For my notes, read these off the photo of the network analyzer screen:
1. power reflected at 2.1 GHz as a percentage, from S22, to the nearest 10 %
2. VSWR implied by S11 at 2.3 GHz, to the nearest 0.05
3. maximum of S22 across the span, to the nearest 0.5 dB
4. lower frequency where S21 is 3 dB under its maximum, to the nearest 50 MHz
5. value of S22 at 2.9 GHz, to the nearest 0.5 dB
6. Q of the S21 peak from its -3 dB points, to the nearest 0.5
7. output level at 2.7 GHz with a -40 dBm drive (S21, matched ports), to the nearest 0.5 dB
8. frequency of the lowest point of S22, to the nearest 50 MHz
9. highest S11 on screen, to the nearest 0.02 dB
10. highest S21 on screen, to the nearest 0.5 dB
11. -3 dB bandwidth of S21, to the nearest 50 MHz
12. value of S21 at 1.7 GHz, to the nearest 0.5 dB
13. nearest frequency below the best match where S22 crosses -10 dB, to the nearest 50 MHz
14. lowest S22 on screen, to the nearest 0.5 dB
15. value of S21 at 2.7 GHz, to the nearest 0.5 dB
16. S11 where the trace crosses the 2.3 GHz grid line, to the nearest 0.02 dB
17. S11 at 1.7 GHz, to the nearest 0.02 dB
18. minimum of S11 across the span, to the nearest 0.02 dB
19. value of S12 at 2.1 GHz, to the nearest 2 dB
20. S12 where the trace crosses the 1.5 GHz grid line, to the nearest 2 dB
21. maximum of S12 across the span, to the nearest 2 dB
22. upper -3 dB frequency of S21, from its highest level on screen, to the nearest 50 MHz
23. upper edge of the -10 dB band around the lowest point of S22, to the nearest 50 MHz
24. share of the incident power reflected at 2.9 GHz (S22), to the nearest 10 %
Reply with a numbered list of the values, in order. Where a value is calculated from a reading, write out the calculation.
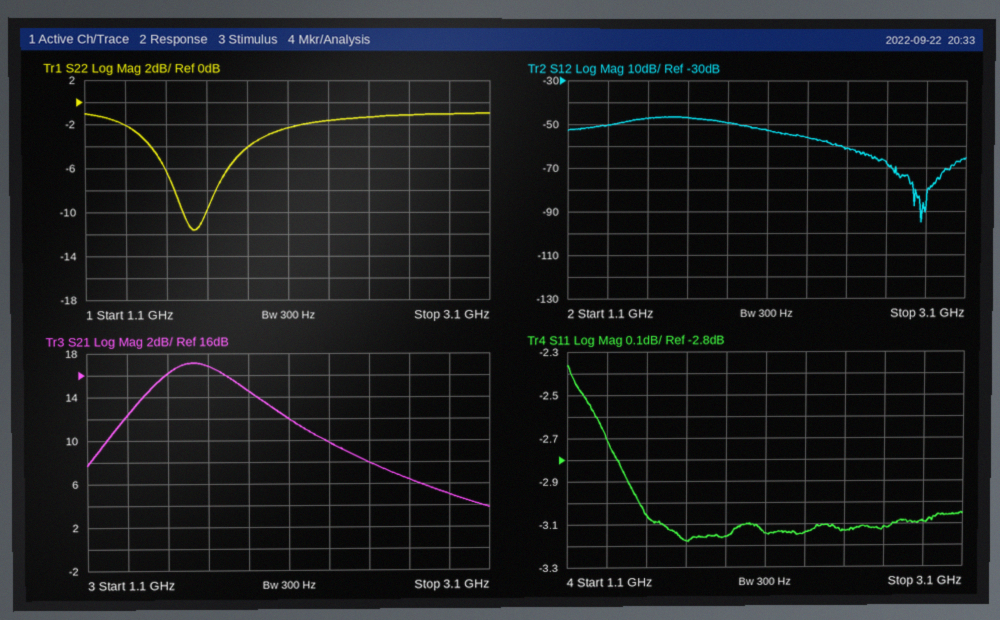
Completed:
1. 10^(-2.5/10) ≈ 56.2 %, so 60 % to the nearest 10 %
2. |Γ| = 10^(-3.14/20) = 0.6966; VSWR = (1 + 0.6966)/(1 − 0.6966) ≈ 5.59, so 5.60 to the nearest 0.05
3. -1.0 dB
4. 1.40 GHz
5. -1.0 dB
6. 1.675 GHz / 550 MHz ≈ 3.0
7. -40 dBm + (6.5 dB) = -33.5 dBm
8. 1.65 GHz
9. -2.36 dB
10. 17.0 dB
11. 1.95 GHz − 1.40 GHz = 550 MHz
12. 17.0 dB
13. 1.60 GHz
14. -11.5 dB
15. 6.5 dB
16. -3.14 dB
17. -3.18 dB
18. -3.18 dB
19. -52 dB
20. -48 dB
21. -46 dB
22. 1.95 GHz
23. 1.70 GHz
24. 10^(-1/10) ≈ 79.4 %, so 80 % to the nearest 10 %
